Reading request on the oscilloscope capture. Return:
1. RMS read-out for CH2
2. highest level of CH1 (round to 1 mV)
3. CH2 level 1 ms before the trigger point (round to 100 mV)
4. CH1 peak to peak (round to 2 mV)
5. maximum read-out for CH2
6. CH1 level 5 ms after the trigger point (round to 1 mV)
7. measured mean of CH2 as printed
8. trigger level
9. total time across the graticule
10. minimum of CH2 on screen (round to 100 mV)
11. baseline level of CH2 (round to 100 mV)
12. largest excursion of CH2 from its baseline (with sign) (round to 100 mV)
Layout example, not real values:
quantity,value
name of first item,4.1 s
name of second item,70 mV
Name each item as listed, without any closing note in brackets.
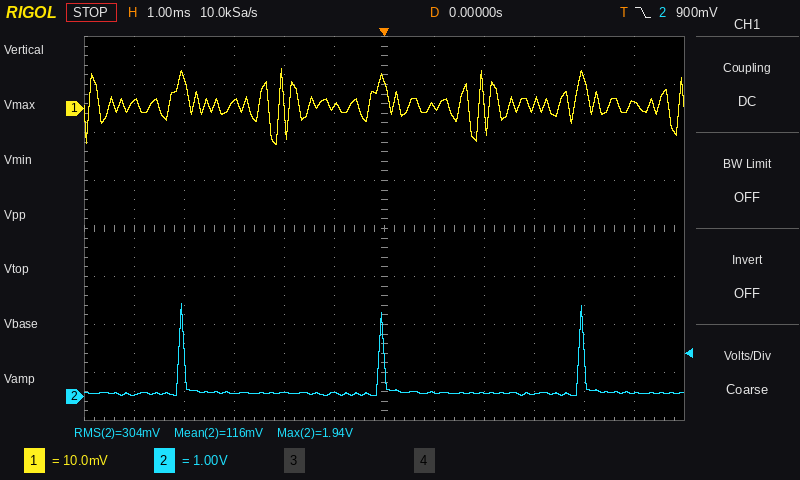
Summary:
quantity,value
RMS read-out for CH2,304 mV
highest level of CH1,8 mV
CH2 level 1 ms before the trigger point,100 mV
CH1 peak to peak,16 mV
maximum read-out for CH2,1.94 V
CH1 level 5 ms after the trigger point,1 mV
measured mean of CH2 as printed,116 mV
trigger level,900 mV
total time across the graticule,12 ms
minimum of CH2 on screen,0.0 V
baseline level of CH2,100 mV
largest excursion of CH2 from its baseline (with sign),+1.9 V
